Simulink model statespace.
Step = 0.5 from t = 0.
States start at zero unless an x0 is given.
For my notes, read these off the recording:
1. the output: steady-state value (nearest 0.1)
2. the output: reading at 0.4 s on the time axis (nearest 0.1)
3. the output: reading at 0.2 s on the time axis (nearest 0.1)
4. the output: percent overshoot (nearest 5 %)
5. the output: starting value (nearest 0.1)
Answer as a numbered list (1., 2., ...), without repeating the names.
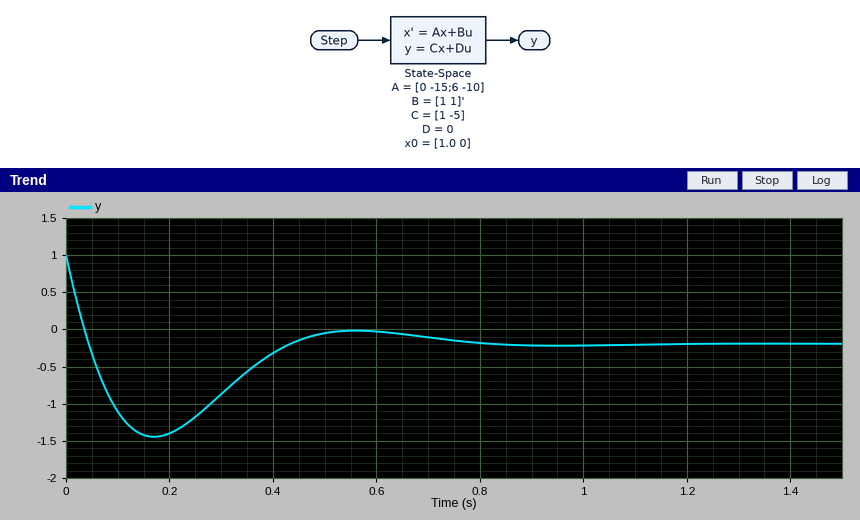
1. -0.2
2. -0.3
3. -1.4
4. 105 %
5. 1.0
